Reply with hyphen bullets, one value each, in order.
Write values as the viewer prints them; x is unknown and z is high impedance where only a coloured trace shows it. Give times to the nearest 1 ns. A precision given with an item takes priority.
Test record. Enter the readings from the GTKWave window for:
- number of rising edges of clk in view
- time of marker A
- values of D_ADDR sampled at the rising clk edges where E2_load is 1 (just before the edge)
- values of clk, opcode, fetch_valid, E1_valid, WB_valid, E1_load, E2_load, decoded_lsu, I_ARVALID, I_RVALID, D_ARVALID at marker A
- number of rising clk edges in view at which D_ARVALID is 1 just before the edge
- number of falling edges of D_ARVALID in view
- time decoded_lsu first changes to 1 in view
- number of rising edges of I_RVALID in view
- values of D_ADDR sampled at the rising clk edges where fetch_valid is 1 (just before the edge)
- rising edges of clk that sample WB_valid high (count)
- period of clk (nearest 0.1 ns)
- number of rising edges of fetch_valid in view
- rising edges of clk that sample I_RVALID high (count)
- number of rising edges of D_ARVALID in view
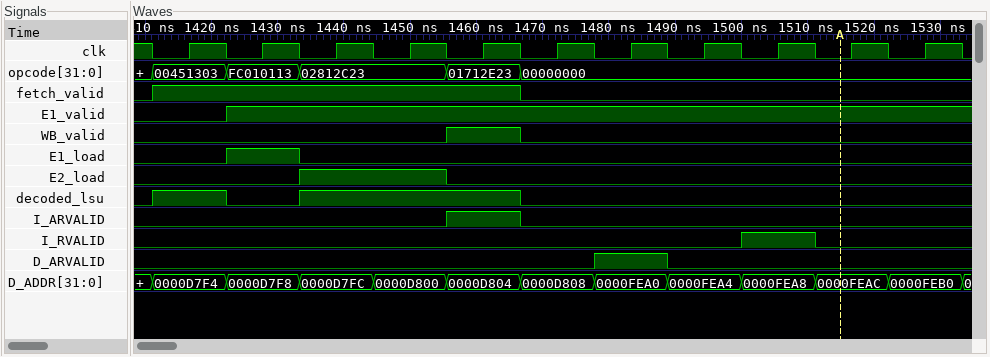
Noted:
- 11
- 1515 ns
- 0000D7FC, 0000D800
- clk=0, opcode=00000000, fetch_valid=0, E1_valid=1, WB_valid=0, E1_load=0, E2_load=0, decoded_lsu=0, I_ARVALID=0, I_RVALID=0, D_ARVALID=0
- 1
- 1
- 1411 ns
- 1
- 0000D7F4, 0000D7F8, 0000D7FC, 0000D800, 0000D804
- 1
- 11.1 ns
- 1
- 1
- 1
